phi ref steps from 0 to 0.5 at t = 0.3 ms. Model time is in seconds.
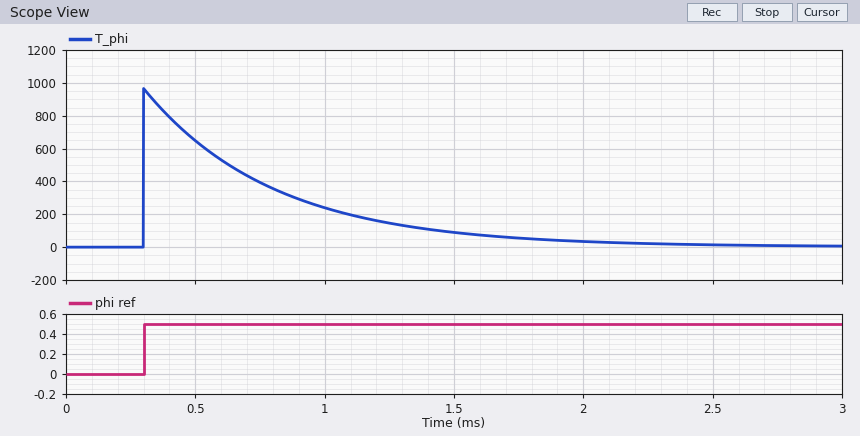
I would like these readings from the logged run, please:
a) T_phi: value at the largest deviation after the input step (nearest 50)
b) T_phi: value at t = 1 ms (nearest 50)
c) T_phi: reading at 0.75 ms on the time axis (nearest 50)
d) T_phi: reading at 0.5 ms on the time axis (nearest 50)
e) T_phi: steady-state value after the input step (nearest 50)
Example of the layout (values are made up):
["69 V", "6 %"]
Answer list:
["950", "250", "400", "650", "0"]
